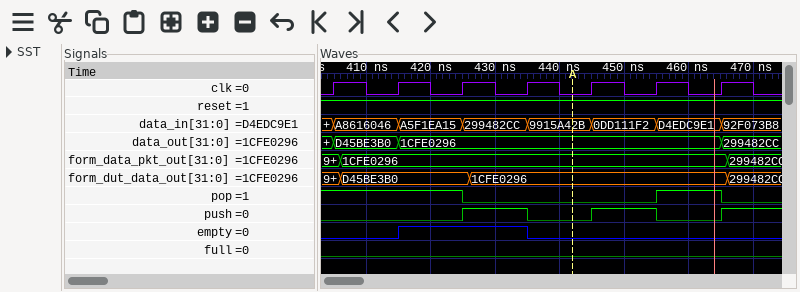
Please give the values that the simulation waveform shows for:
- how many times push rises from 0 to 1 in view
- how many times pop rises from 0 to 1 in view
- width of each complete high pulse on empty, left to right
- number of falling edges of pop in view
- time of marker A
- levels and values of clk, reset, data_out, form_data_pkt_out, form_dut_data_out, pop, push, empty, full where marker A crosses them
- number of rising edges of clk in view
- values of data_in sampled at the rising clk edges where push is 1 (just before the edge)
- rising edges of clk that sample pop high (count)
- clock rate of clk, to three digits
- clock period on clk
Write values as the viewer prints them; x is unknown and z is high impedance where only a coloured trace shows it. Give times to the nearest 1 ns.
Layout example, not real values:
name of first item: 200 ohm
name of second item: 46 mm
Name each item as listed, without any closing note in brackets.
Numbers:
how many times push rises from 0 to 1 in view: 3
how many times pop rises from 0 to 1 in view: 1
width of each complete high pulse on empty, left to right: 20 ns
number of falling edges of pop in view: 2
time of marker A: 442 ns
levels and values of clk, reset, data_out, form_data_pkt_out, form_dut_data_out, pop, push, empty, full where marker A crosses them: clk=0, reset=1, data_out=1CFE0296, form_data_pkt_out=1CFE0296, form_dut_data_out=1CFE0296, pop=0, push=0, empty=0, full=0
number of rising edges of clk in view: 7
values of data_in sampled at the rising clk edges where push is 1: 299482CC, 0DD111F2
rising edges of clk that sample pop high: 4
clock rate of clk, to three digits: 100 MHz
clock period on clk: 10 ns
